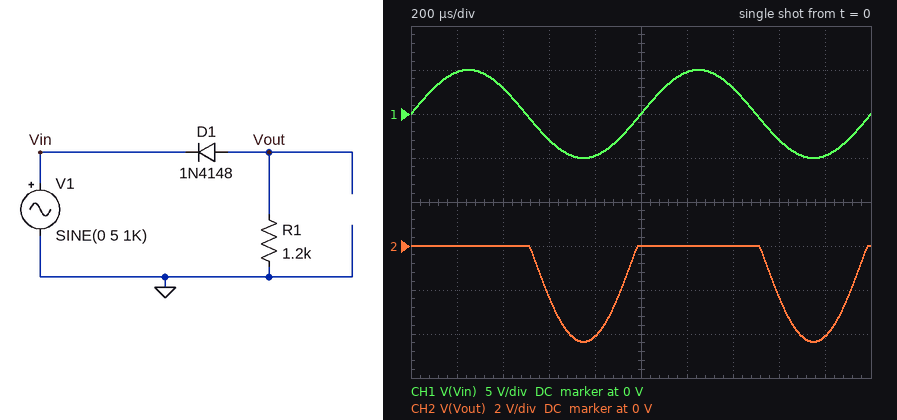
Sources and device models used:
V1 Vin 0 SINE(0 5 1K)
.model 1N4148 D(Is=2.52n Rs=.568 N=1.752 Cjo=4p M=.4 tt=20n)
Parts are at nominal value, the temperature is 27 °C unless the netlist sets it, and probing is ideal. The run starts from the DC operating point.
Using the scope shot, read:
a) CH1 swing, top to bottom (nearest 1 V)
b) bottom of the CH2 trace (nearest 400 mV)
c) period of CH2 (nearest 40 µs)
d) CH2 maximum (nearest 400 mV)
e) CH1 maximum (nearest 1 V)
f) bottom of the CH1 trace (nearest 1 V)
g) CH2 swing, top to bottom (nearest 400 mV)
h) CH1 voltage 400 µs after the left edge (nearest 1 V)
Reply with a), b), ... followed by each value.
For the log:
a) 10 V
b) -4.4 V
c) 1.00 ms
d) 0 V
e) 5 V
f) -5 V
g) 4.4 V
h) 3 V
